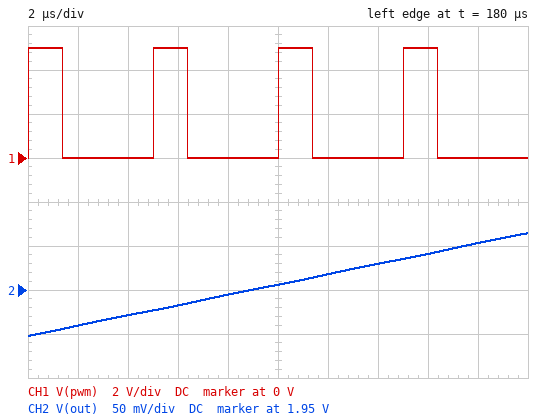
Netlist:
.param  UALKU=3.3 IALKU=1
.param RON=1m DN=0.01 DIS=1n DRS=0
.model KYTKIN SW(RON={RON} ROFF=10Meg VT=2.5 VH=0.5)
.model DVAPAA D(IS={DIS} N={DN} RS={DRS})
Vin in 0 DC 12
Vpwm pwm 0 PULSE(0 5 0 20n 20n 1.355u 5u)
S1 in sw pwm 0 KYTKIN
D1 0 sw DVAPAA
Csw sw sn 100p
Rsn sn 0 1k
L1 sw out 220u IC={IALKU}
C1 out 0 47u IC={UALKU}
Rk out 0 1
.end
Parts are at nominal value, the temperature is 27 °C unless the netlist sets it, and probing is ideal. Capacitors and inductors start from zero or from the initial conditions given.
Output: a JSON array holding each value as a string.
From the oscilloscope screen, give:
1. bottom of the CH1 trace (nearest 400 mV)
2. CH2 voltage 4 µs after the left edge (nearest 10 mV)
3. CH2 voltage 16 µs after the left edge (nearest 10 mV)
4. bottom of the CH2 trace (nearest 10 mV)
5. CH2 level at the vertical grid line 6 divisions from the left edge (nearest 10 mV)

["0 V", "1.92 V", "1.99 V", "1.90 V", "1.97 V"]
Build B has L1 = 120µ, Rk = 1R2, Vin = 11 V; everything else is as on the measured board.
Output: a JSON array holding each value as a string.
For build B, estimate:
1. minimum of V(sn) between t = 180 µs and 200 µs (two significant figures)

["-11 V"]
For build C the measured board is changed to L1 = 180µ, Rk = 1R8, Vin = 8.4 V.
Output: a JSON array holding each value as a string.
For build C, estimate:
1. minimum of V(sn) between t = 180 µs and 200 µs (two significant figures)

["-8.4 V"]
